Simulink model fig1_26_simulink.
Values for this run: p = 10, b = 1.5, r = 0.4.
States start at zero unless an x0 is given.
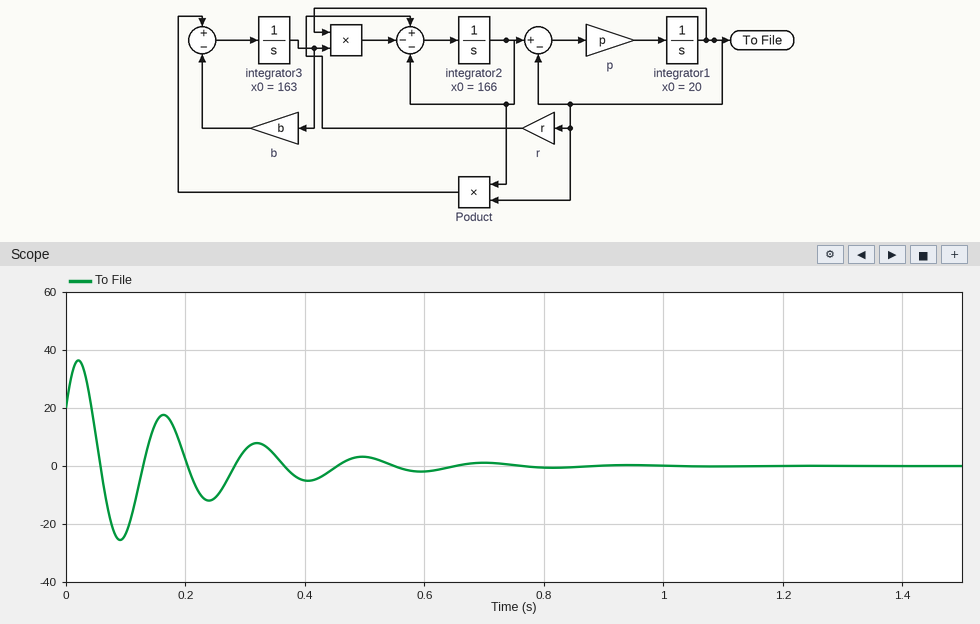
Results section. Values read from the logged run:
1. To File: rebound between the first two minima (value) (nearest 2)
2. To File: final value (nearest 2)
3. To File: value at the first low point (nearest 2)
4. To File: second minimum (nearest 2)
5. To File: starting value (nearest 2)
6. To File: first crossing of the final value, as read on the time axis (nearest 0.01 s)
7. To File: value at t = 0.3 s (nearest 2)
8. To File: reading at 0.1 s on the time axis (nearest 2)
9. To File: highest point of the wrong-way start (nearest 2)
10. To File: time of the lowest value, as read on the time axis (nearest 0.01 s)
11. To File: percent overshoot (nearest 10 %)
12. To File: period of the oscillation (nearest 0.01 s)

18
0
-26
-12
20
0.06 s
6
-24
36
0.09 s
130 %
0.15 s
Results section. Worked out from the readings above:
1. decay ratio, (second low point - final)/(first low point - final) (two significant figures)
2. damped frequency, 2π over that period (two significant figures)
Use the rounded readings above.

0.46
42 rad/s
